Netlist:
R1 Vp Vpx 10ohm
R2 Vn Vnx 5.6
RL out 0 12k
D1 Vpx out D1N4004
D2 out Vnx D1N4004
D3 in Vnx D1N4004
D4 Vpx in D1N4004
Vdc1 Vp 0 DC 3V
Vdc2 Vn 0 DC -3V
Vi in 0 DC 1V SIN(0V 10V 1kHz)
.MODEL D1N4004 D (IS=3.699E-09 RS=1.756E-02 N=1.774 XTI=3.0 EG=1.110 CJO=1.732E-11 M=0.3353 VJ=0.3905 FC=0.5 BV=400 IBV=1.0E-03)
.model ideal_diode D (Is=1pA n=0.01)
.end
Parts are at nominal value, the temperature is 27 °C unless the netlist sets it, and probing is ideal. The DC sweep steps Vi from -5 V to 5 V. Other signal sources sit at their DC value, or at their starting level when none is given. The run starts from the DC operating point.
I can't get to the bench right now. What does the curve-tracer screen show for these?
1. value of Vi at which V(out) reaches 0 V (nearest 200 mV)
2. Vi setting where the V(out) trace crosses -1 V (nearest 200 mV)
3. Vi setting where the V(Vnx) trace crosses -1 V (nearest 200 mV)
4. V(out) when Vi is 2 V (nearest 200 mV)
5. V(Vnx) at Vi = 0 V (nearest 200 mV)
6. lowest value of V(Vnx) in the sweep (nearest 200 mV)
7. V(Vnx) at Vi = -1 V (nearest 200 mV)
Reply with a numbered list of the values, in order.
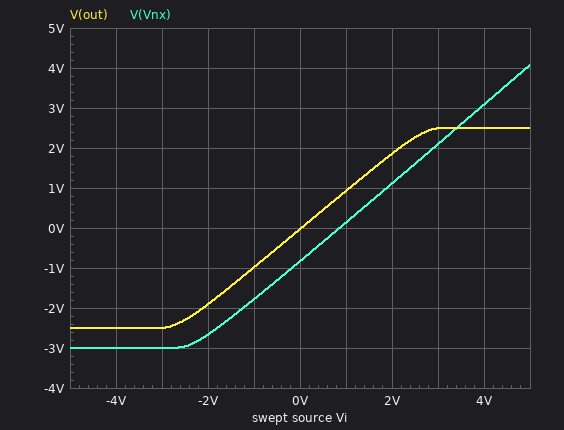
1. 0 V
2. -1.0 V
3. -200 mV
4. 1.8 V
5. -800 mV
6. -3.0 V
7. -1.8 V
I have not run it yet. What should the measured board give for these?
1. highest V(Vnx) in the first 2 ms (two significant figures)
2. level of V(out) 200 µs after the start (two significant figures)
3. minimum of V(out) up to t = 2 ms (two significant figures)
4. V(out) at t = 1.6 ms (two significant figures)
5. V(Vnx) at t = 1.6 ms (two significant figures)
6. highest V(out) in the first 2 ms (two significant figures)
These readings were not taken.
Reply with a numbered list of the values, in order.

1. 9.0 V
2. 2.5 V
3. -2.5 V
4. -2.5 V
5. -3.0 V
6. 2.5 V
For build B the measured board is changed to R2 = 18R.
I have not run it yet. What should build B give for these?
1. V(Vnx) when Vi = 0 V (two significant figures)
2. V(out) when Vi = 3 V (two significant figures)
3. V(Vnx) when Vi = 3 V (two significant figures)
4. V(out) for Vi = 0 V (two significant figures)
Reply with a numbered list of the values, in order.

1. -750 mV
2. 2.5 V
3. 2.2 V
4. 27 mV
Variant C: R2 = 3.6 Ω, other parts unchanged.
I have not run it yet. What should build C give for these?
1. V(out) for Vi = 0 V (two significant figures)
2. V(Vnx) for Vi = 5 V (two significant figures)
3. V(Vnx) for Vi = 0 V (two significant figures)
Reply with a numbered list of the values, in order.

1. -49 mV
2. 4.0 V
3. -860 mV
